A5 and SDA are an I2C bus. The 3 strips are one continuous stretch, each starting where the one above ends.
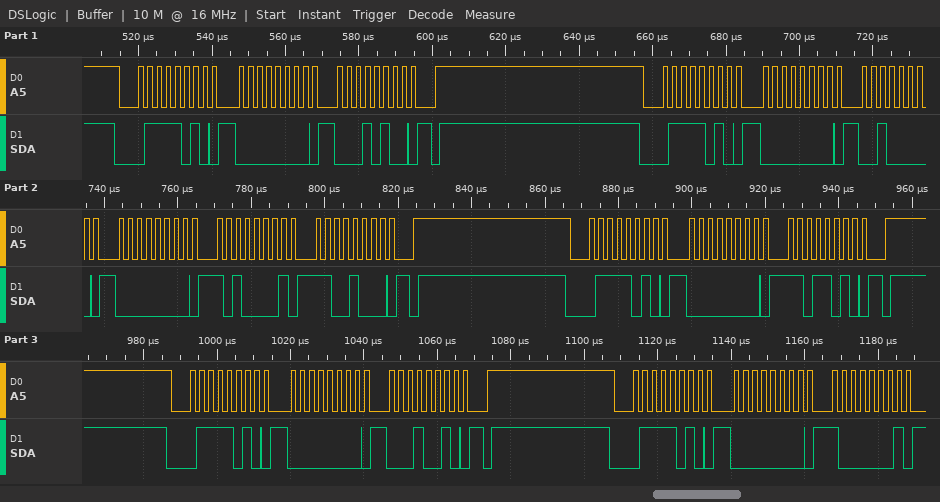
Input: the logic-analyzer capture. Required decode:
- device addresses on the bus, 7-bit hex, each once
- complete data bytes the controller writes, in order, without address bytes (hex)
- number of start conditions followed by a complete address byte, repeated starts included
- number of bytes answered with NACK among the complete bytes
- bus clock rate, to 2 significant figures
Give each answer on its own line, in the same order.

0x3D
00 14 00 20 00 A1 C8 00 DA 00 12 00 81
5
0
400 kHz
